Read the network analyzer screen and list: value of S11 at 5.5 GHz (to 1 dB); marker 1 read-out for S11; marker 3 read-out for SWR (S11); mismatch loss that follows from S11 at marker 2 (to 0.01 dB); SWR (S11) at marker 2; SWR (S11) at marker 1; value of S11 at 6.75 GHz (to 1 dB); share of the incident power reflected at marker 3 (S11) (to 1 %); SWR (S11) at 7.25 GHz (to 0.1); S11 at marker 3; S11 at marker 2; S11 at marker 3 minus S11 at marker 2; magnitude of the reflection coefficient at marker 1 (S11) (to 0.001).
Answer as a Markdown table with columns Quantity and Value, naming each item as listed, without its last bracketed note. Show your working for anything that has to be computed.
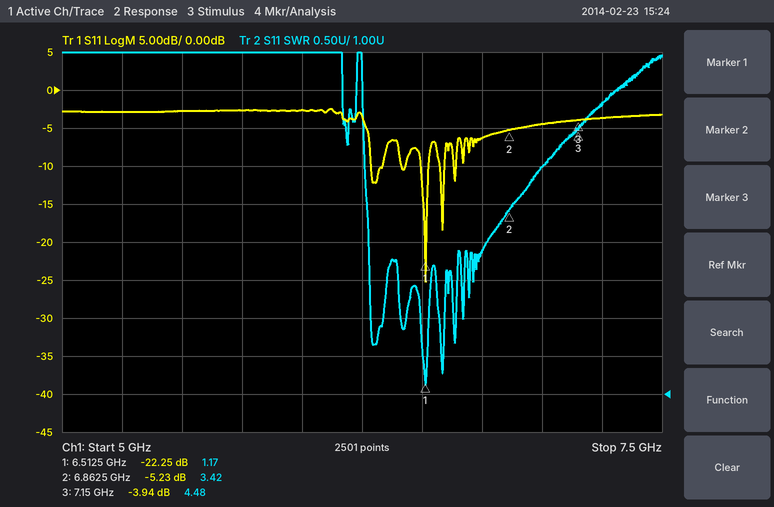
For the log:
| Quantity | Value |
|---|---|
| value of S11 at 5.5 GHz | -3 dB |
| marker 1 read-out for S11 | -22.25 dB |
| marker 3 read-out for SWR | 4.48 |
| mismatch loss that follows from S11 at marker 2 | −10 log10(1 − 10^(-5.23/10)) ≈ 1.55 dB |
| SWR (S11) at marker 2 | 3.42 |
| SWR (S11) at marker 1 | 1.17 |
| value of S11 at 6.75 GHz | -6 dB |
| share of the incident power reflected at marker 3 (S11) | 10^(-3.94/10) ≈ 40 % |
| SWR (S11) at 7.25 GHz | 4.8 |
| S11 at marker 3 | -3.94 dB |
| S11 at marker 2 | -5.23 dB |
| S11 at marker 3 minus S11 at marker 2 | -3.94 − (-5.23) = 1.29 dB |
| magnitude of the reflection coefficient at marker 1 (S11) | 10^(-22.25/20) ≈ 0.077 |
